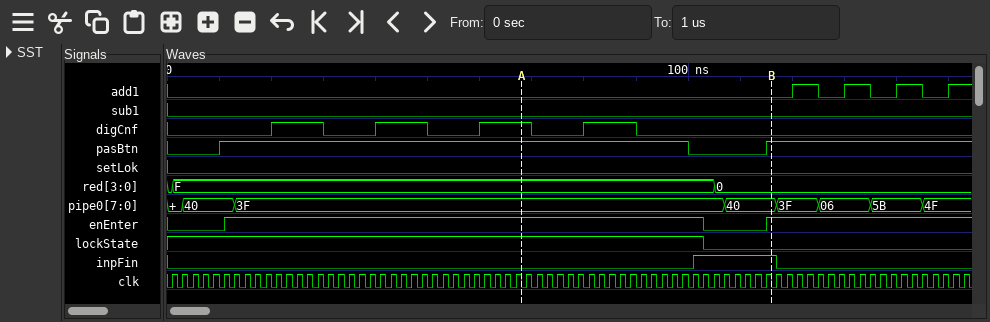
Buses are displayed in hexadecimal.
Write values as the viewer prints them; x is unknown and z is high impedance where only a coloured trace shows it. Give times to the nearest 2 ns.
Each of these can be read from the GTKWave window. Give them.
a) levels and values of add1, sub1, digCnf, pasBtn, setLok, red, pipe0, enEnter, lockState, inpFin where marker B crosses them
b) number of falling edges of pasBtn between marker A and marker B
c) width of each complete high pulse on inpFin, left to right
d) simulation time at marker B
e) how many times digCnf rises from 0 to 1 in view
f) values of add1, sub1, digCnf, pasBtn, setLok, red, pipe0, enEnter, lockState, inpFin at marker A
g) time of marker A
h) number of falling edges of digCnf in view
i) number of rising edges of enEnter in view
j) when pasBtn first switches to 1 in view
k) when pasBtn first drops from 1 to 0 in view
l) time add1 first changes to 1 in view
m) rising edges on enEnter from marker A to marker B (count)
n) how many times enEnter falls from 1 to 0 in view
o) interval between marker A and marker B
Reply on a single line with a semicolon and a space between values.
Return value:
add1=0, sub1=0, digCnf=0, pasBtn=1, setLok=0, red=0, pipe0=40, enEnter=1, lockState=0, inpFin=1; 1; 16 ns; 116 ns; 4; add1=0, sub1=0, digCnf=1, pasBtn=1, setLok=0, red=F, pipe0=3F, enEnter=1, lockState=1, inpFin=0; 68 ns; 4; 2; 10 ns; 100 ns; 120 ns; 1; 1; 48 ns
